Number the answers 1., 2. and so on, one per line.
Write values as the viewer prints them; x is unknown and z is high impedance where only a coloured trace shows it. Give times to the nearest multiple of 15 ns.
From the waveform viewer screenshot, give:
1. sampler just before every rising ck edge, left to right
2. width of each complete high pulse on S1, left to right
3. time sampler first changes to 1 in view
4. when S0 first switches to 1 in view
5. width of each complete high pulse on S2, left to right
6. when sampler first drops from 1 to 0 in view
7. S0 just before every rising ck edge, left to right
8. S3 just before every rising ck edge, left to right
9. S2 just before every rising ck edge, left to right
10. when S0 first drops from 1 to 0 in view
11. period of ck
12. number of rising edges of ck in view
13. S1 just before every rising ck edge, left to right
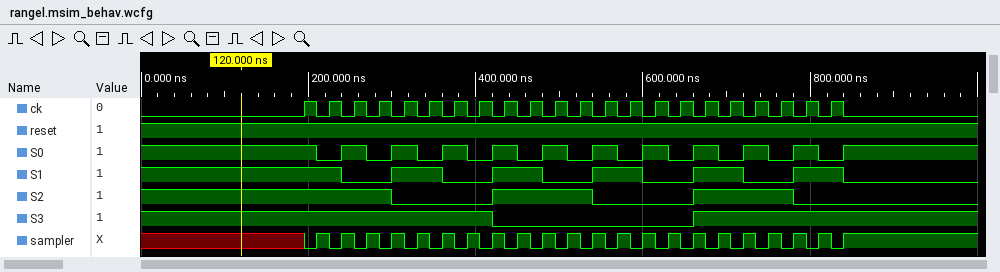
1. x 1 1 1 1 1 1 1 1 1 1 1 1 1 1 1 1 1 1 1 1 1
2. 60 ns, 60 ns, 60 ns, 60 ns, 60 ns
3. 210 ns
4. 240 ns
5. 120 ns, 120 ns
6. 225 ns
7. 1 0 1 0 1 0 1 0 1 0 1 0 1 0 1 0 1 0 1 0 1 0
8. 1 1 1 1 1 1 1 1 0 0 0 0 0 0 0 0 1 1 1 1 1 1
9. 1 1 1 1 0 0 0 0 1 1 1 1 0 0 0 0 1 1 1 1 0 0
10. 210 ns
11. 30 ns
12. 22
13. 1 1 0 0 1 1 0 0 1 1 0 0 1 1 0 0 1 1 0 0 1 1
